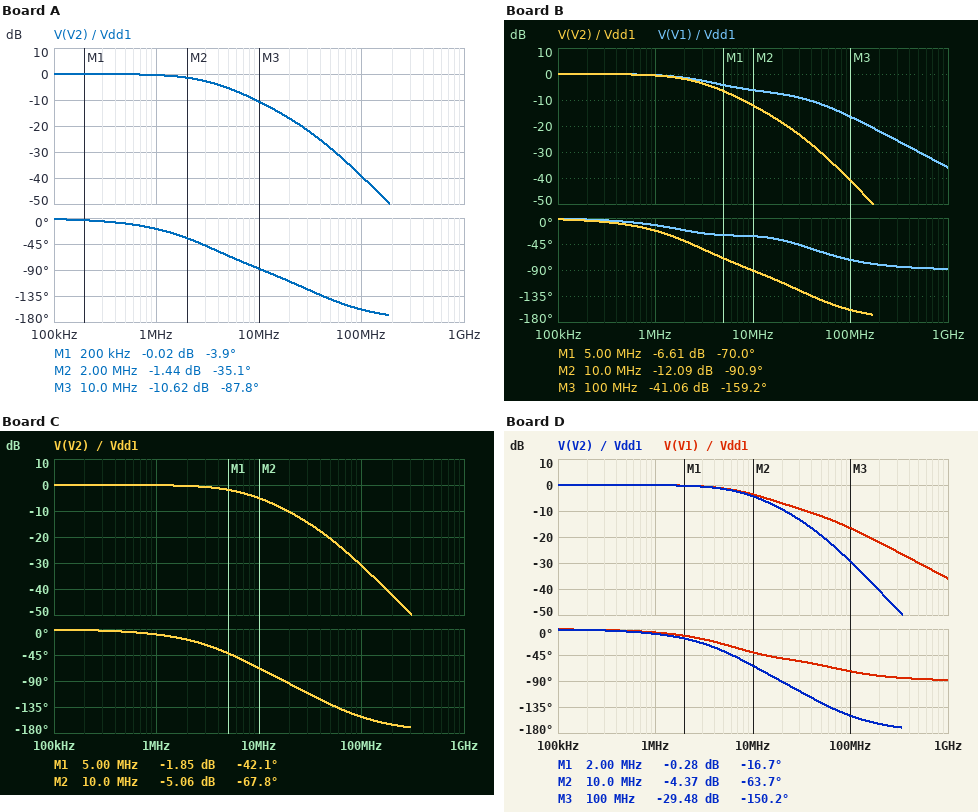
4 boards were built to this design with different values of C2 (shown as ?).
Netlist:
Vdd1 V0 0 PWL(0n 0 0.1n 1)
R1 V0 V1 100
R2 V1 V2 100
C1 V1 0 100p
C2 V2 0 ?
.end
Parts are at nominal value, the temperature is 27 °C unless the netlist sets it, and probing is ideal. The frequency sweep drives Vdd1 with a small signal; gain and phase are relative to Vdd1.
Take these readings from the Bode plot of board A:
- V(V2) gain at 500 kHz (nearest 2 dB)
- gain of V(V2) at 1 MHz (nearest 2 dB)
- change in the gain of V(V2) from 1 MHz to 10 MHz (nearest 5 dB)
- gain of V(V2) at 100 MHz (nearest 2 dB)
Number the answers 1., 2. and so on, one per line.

1. 0 dB
2. 0 dB
3. -10 dB
4. -40 dB
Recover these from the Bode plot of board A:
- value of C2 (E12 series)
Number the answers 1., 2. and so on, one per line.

1. 220 pF
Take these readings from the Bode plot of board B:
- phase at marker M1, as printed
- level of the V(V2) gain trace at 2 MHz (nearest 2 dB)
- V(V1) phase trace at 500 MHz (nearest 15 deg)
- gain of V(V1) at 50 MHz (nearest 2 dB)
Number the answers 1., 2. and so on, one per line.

1. -70.0 deg
2. -2 dB
3. -90 deg
4. -12 dB
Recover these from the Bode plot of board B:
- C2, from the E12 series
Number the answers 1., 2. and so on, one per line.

1. 270 pF
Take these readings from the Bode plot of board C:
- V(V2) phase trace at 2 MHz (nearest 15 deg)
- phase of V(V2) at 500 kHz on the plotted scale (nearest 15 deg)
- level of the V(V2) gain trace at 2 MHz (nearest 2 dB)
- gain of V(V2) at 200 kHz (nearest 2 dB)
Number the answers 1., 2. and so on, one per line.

1. -15 deg
2. 0 deg
3. 0 dB
4. 0 dB
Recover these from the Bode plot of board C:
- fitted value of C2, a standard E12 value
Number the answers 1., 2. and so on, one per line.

1. 82 pF
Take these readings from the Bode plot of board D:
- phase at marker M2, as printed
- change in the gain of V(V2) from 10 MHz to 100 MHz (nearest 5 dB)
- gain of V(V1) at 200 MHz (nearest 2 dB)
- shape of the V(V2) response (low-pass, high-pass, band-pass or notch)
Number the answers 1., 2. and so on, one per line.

1. -63.7 deg
2. -25 dB
3. -22 dB
4. low-pass
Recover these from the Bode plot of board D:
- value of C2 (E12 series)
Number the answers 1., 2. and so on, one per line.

1. 68 pF
